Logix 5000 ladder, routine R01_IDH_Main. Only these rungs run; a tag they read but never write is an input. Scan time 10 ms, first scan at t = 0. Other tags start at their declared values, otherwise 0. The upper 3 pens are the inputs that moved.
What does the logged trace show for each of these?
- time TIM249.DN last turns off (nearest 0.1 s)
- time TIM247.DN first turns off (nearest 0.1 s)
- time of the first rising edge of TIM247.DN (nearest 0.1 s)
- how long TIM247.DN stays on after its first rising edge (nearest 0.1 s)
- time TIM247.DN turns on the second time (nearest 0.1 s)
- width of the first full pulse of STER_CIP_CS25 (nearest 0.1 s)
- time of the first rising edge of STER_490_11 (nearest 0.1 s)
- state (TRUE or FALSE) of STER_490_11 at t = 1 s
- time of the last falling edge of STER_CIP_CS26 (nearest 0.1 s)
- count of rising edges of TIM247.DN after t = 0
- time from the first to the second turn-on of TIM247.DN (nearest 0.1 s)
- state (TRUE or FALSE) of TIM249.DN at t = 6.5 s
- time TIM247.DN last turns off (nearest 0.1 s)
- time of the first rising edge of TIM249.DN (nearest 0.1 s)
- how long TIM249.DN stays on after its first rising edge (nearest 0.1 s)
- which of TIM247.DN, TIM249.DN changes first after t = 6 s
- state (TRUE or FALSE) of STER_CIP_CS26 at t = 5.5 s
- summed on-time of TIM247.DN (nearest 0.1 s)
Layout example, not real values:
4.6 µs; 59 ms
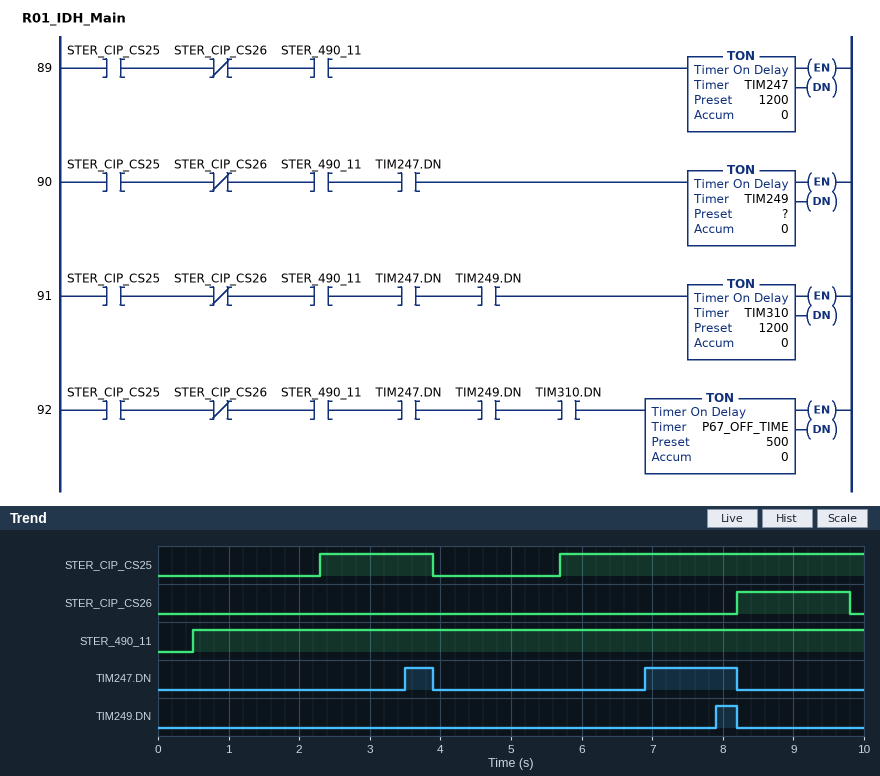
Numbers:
8.2 s; 3.9 s; 3.5 s; 0.4 s; 6.9 s; 1.6 s; 0.5 s; TRUE; 9.8 s; 2; 3.4 s; FALSE; 8.2 s; 7.9 s; 0.3 s; TIM247.DN; FALSE; 1.7 s
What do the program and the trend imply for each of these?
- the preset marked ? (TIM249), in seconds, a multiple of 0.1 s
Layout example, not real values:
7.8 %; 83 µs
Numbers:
1.0 s
